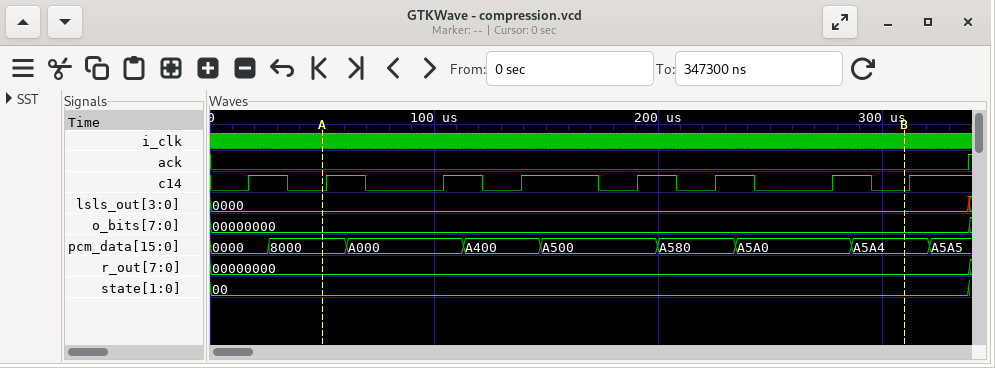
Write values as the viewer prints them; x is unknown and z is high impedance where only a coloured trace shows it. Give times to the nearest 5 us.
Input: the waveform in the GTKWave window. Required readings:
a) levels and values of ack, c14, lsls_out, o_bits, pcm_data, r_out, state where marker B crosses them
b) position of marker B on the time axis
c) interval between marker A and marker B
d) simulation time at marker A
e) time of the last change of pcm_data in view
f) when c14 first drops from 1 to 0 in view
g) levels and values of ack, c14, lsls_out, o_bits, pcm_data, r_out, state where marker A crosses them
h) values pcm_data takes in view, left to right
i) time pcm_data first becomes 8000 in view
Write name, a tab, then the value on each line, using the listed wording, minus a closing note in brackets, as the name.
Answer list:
levels and values of ack, c14, lsls_out, o_bits, pcm_data, r_out, state where marker B crosses them	ack=0, c14=0, lsls_out=0000, o_bits=00000000, pcm_data=A5A4, r_out=00000000, state=00
position of marker B on the time axis	310 us
interval between marker A and marker B	260 us
simulation time at marker A	50 us
time of the last change of pcm_data in view	320 us
when c14 first drops from 1 to 0 in view	35 us
levels and values of ack, c14, lsls_out, o_bits, pcm_data, r_out, state where marker A crosses them	ack=0, c14=0, lsls_out=0000, o_bits=00000000, pcm_data=8000, r_out=00000000, state=00
values pcm_data takes in view, left to right	0000, 8000, A000, A400, A500, A580, A5A0, A5A4, A5A5
time pcm_data first becomes 8000 in view	25 us
